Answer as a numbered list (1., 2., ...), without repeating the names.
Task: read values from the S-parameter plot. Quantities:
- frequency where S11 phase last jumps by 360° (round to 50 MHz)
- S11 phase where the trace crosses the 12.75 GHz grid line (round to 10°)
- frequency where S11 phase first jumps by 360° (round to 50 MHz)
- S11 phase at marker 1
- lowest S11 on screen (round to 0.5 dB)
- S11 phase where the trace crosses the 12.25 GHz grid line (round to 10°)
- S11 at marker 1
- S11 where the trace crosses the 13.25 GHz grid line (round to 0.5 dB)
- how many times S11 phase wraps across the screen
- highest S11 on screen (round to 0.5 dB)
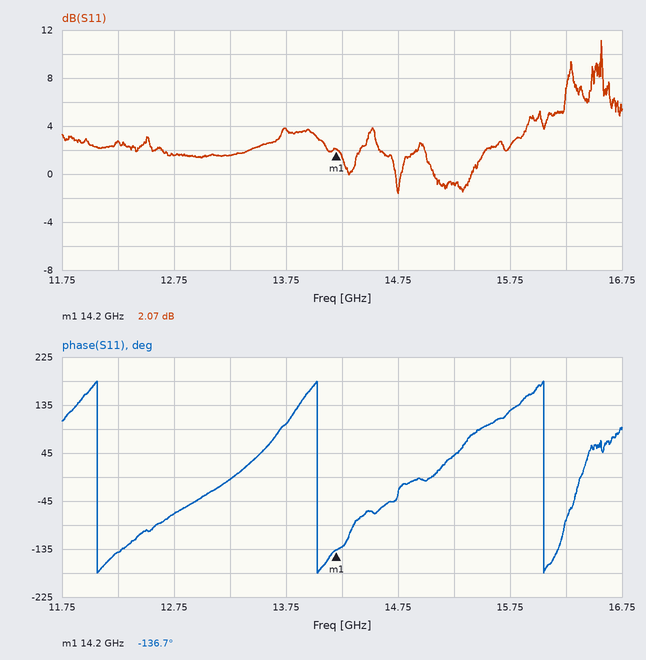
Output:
1. 16.05 GHz
2. -70°
3. 12.05 GHz
4. -136.7°
5. -1.5 dB
6. -140°
7. 2.07 dB
8. 1.5 dB
9. 3
10. 11.0 dB
